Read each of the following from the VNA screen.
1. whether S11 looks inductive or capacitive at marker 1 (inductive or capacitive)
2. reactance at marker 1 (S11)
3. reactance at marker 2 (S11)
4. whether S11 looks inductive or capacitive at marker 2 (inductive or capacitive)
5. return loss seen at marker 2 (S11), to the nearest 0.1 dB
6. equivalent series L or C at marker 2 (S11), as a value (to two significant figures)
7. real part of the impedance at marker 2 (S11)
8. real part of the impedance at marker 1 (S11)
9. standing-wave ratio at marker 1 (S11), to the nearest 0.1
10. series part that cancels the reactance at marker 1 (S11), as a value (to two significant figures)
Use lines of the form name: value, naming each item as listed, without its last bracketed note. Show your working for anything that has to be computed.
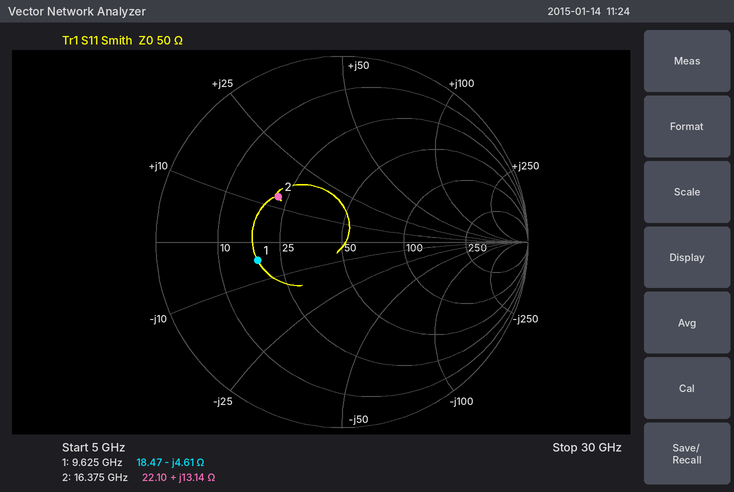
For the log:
whether S11 looks inductive or capacitive at marker 1: capacitive
reactance at marker 1: -4.61 Ω
reactance at marker 2: +13.14 Ω
whether S11 looks inductive or capacitive at marker 2: inductive
return loss seen at marker 2 (S11), to the nearest 0.1 dB: 7.5 dB
equivalent series L or C at marker 2 (S11), as a value: L = 13.14 Ω/(2π × 16.375 GHz) ≈ 128 pH, so 130 pH to two significant figures
real part of the impedance at marker 2: 22.10 Ω
real part of the impedance at marker 1: 18.47 Ω
standing-wave ratio at marker 1 (S11), to the nearest 0.1: 2.7
series part that cancels the reactance at marker 1 (S11), as a value: L = 4.61 Ω/(2π × 9.625 GHz) ≈ 76 pH
